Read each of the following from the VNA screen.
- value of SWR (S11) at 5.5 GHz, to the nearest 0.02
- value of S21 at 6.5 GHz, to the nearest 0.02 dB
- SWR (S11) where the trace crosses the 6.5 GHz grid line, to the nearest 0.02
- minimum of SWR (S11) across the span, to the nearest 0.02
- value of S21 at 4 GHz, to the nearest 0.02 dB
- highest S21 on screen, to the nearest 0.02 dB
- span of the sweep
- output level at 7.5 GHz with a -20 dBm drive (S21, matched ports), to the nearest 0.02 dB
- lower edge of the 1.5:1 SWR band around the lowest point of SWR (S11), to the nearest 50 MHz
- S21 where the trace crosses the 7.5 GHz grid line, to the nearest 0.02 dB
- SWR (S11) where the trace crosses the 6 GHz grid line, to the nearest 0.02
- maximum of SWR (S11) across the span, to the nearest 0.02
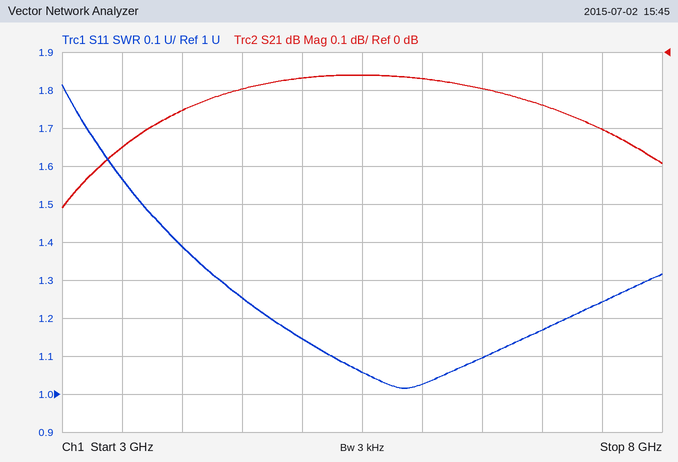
1.06
-0.10 dB
1.10
1.02
-0.16 dB
-0.06 dB
5 GHz
-20.20 dBm
3.65 GHz
-0.20 dB
1.02
1.82
